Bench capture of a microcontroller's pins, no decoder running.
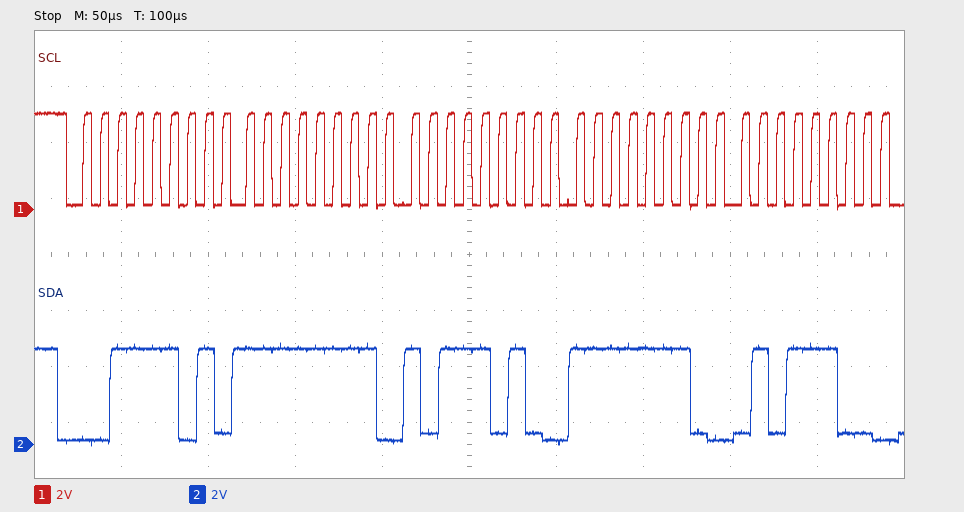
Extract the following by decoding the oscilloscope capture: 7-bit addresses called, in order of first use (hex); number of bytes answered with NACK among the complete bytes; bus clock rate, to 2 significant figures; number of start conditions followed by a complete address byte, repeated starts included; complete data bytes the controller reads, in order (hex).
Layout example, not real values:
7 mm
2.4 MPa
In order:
0x1E
0
100 kHz
1
FF BA FE 5C
